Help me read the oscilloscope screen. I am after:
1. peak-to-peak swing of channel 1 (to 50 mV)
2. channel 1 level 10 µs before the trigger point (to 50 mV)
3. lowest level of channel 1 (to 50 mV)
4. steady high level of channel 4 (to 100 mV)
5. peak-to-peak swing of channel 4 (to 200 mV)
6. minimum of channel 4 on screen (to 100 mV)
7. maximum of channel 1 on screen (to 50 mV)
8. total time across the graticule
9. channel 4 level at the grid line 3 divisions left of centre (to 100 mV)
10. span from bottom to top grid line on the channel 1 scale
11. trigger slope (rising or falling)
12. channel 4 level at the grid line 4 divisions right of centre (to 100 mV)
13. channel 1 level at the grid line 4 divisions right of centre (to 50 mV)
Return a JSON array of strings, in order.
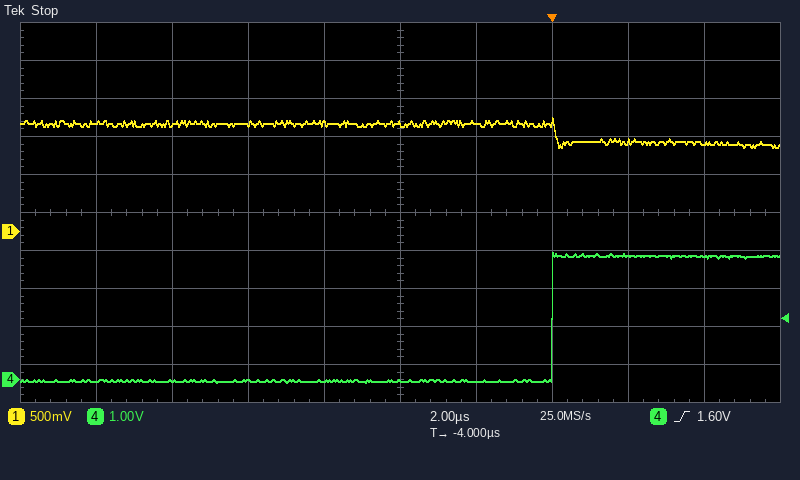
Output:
["400 mV", "1.40 V", "1.10 V", "3.3 V", "3.4 V", "-100 mV", "1.50 V", "20 µs", "0.0 V", "5 V", "rising", "3.2 V", "1.15 V"]
